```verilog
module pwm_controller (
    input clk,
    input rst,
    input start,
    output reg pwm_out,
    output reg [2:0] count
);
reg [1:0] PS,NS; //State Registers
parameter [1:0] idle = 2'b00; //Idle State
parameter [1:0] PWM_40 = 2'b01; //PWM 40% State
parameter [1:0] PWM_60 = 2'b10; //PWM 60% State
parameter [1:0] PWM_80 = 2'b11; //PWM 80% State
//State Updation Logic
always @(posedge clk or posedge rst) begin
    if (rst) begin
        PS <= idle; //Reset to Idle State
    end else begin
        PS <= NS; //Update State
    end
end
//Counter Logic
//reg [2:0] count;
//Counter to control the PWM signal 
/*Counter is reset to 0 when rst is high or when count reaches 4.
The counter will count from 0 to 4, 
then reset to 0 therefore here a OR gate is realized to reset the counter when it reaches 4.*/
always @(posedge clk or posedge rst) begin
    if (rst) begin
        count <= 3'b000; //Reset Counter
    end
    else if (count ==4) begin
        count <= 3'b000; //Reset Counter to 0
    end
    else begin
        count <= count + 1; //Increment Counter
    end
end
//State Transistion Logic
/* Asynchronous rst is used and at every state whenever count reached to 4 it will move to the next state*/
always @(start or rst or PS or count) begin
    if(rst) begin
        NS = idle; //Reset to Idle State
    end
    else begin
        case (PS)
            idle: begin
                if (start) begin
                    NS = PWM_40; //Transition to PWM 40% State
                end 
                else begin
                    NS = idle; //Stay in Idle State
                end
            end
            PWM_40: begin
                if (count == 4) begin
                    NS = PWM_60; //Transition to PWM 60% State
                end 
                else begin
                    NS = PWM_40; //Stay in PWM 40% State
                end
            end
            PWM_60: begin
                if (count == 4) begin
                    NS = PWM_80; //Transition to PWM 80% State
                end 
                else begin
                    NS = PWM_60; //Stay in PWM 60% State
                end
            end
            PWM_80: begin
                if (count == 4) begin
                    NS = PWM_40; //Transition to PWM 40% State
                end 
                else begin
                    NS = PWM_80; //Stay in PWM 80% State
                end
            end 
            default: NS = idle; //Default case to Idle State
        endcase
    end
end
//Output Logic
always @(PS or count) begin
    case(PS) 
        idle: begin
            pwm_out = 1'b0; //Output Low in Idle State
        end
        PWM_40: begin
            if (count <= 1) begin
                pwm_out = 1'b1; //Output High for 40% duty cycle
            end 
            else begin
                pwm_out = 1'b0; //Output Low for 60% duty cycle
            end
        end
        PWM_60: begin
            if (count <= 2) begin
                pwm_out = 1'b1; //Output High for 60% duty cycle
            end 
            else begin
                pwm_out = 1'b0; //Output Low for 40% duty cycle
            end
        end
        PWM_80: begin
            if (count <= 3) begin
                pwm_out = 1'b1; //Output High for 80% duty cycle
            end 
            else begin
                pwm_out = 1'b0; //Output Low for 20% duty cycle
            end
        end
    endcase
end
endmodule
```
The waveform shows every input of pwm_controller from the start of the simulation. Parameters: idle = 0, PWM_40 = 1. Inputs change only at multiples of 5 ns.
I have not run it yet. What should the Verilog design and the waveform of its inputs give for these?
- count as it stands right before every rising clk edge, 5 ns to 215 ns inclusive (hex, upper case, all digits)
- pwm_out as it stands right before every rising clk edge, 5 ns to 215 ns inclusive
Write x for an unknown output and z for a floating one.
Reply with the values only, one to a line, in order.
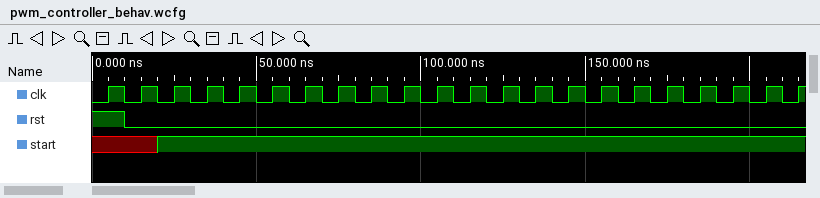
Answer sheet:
0, 0, 1, 2, 3, 4, 0, 1, 2, 3, 4, 0, 1, 2, 3, 4, 0, 1, 2, 3, 4, 0
0 0 0 0 0 0 1 1 1 0 0 1 1 1 1 0 1 1 0 0 0 1
